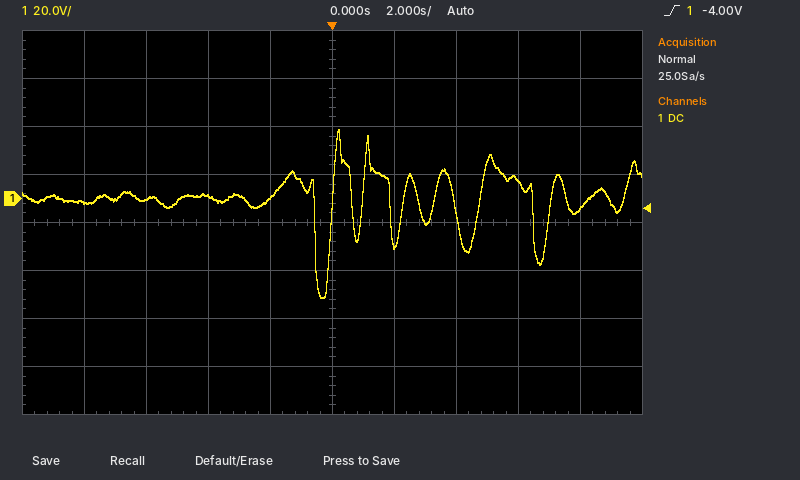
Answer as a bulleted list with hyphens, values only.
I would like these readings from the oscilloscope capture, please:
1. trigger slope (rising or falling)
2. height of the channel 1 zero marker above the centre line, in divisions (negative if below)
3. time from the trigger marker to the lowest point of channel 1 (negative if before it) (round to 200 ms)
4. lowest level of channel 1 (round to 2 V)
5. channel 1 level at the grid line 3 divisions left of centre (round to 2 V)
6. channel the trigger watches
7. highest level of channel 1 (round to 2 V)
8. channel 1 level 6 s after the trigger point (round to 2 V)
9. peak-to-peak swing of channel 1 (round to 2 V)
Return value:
- rising
- +0.5 div
- -400 ms
- -42 V
- 0 V
- channel 1
- 28 V
- 8 V
- 70 V
